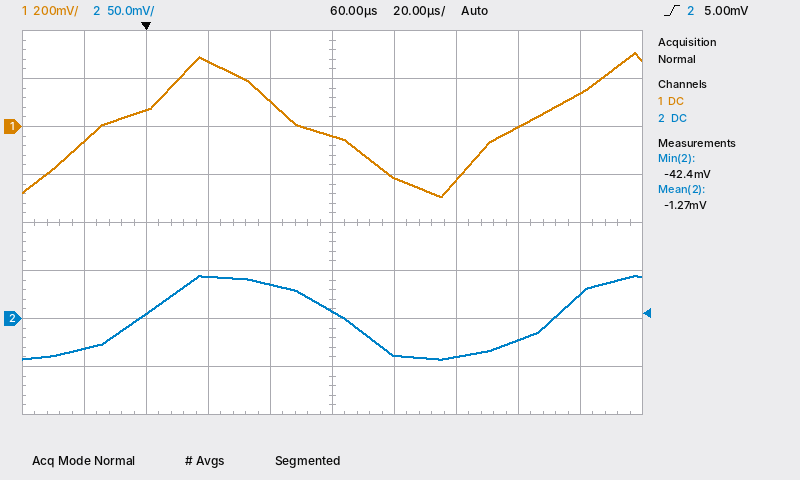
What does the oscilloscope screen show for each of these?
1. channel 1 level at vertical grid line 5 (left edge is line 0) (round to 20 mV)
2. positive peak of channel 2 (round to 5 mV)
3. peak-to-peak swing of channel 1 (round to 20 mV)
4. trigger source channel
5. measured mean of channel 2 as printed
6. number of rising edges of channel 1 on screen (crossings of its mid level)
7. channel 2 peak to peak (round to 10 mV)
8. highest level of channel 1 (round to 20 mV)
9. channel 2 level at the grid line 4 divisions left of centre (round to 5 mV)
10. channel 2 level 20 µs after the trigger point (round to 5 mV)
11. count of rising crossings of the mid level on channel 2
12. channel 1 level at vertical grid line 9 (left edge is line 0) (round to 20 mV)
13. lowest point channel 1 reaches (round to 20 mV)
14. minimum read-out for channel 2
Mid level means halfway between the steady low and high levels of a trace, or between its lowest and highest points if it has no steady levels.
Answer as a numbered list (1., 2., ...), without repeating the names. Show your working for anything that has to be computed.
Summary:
1. -40 mV
2. 45 mV
3. 300 mV − (-300 mV) = 600 mV
4. channel 2
5. -1.27 mV
6. 2
7. 90 mV
8. 300 mV
9. -30 mV
10. 45 mV
11. 2
12. 140 mV
13. -300 mV
14. -42.4 mV
